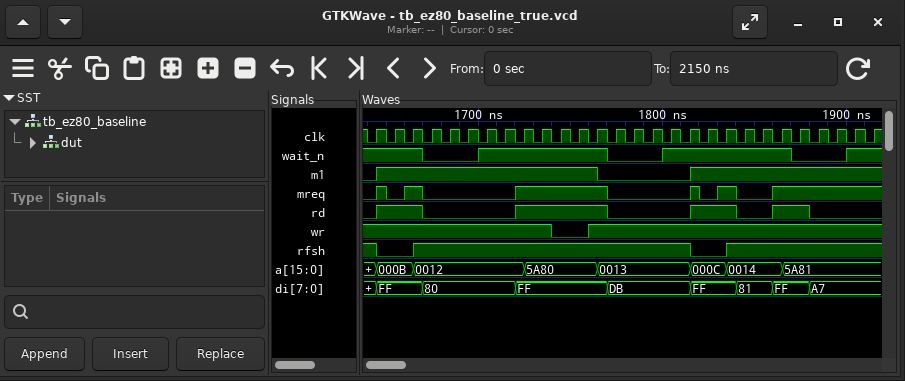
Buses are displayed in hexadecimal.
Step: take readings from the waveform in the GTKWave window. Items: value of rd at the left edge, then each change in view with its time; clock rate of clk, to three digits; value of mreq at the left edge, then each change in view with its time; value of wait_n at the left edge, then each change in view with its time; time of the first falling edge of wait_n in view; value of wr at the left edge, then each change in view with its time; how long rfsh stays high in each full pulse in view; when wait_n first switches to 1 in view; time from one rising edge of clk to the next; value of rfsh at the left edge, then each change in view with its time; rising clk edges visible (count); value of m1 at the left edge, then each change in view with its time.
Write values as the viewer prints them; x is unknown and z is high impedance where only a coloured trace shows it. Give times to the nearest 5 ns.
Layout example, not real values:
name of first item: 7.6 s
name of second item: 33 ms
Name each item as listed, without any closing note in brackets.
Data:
value of rd at the left edge, then each change in view with its time: 0, 1 at 1645 ns, 0 at 1670 ns, 1 at 1720 ns, 0 at 1770 ns, 1 at 1815 ns, 0 at 1840 ns, 1 at 1860 ns, 0 at 1880 ns
clock rate of clk, to three digits: 100 MHz
value of mreq at the left edge, then each change in view with its time: 0, 1 at 1645 ns, 0 at 1650 ns, 1 at 1660 ns, 0 at 1670 ns, 1 at 1720 ns, 0 at 1770 ns, 1 at 1815 ns, 0 at 1820 ns, 1 at 1830 ns, 0 at 1840 ns, 1 at 1860 ns
value of wait_n at the left edge, then each change in view with its time: 1, 0 at 1670 ns, 1 at 1700 ns, 0 at 1770 ns, 1 at 1800 ns, 0 at 1870 ns, 1 at 1900 ns
time of the first falling edge of wait_n in view: 1670 ns
value of wr at the left edge, then each change in view with its time: 1, 0 at 1740 ns, 1 at 1760 ns
how long rfsh stays high in each full pulse in view: 150 ns
when wait_n first switches to 1 in view: 1700 ns
time from one rising edge of clk to the next: 10 ns
value of rfsh at the left edge, then each change in view with its time: 1, 0 at 1645 ns, 1 at 1665 ns, 0 at 1815 ns, 1 at 1835 ns
rising clk edges visible: 28
value of m1 at the left edge, then each change in view with its time: 0, 1 at 1645 ns, 0 at 1765 ns, 1 at 1815 ns
